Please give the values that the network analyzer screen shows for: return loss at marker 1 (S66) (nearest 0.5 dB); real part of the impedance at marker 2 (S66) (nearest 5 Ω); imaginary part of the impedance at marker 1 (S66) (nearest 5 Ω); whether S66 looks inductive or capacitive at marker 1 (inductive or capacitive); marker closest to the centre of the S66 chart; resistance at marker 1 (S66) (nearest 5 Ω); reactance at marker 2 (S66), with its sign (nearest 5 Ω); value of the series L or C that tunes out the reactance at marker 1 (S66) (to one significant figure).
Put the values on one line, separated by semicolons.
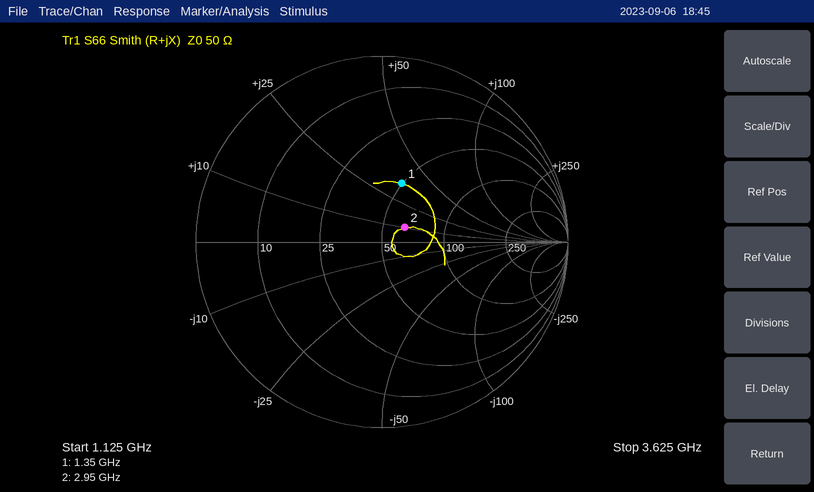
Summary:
9.5 dB; 65 Ω; +35 Ω; inductive; marker 2; 50 Ω; +10 Ω; 3 pF
